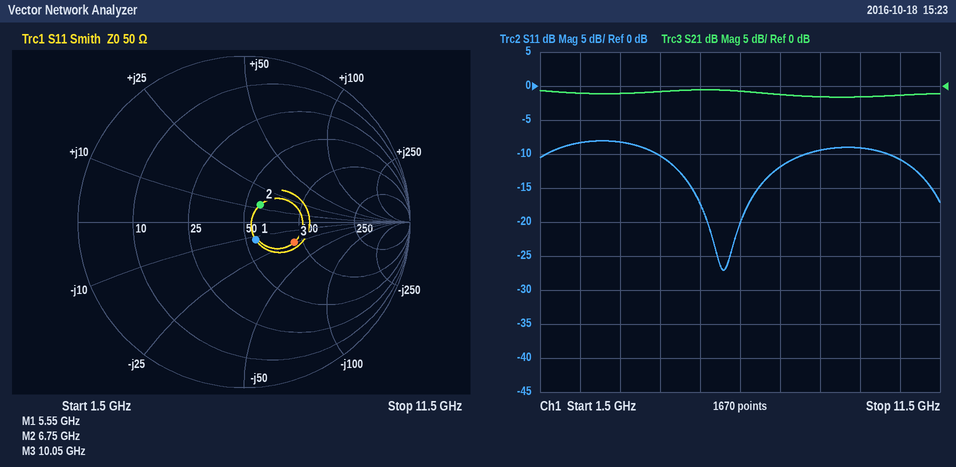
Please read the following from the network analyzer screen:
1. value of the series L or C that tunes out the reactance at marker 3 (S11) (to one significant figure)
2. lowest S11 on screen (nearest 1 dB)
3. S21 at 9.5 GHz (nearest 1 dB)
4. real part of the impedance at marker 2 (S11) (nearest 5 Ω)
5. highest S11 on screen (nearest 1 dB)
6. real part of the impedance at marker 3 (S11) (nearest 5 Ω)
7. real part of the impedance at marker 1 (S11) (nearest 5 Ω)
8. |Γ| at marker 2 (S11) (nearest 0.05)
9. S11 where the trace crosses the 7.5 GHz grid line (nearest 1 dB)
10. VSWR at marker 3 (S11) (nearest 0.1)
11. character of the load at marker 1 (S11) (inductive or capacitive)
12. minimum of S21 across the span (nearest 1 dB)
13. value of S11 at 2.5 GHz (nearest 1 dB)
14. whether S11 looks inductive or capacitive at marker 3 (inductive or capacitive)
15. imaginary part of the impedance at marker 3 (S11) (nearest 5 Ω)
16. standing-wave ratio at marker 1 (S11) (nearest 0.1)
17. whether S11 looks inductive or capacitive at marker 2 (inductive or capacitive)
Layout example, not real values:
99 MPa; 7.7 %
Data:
400 pH; -27 dB; -2 dB; 60 Ω; -8 dB; 90 Ω; 55 Ω; 0.15; -12 dB; 2.0; capacitive; -2 dB; -8 dB; capacitive; -25 Ω; 1.3; inductive
